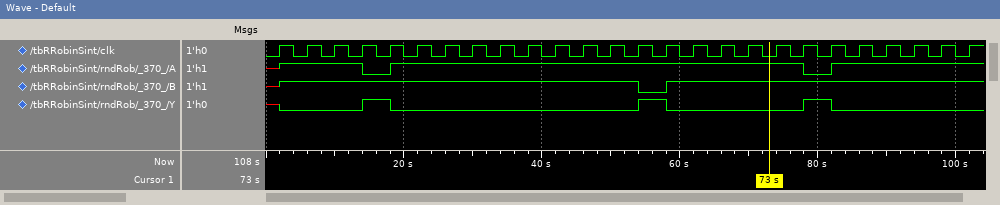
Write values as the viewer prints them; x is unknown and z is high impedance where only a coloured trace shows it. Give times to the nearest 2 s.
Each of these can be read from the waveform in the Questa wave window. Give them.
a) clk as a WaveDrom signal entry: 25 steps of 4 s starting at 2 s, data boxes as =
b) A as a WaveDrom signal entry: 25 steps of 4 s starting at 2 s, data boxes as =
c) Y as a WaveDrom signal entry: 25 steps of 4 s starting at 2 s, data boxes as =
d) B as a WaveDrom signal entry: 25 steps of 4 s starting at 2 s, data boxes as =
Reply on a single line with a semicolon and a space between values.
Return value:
{name: 'clk', wave: 'p........................'}; {name: 'A', wave: '1..01..............01....'}; {name: 'Y', wave: '0..10........10....10....'}; {name: 'B', wave: '1............01..........'}
